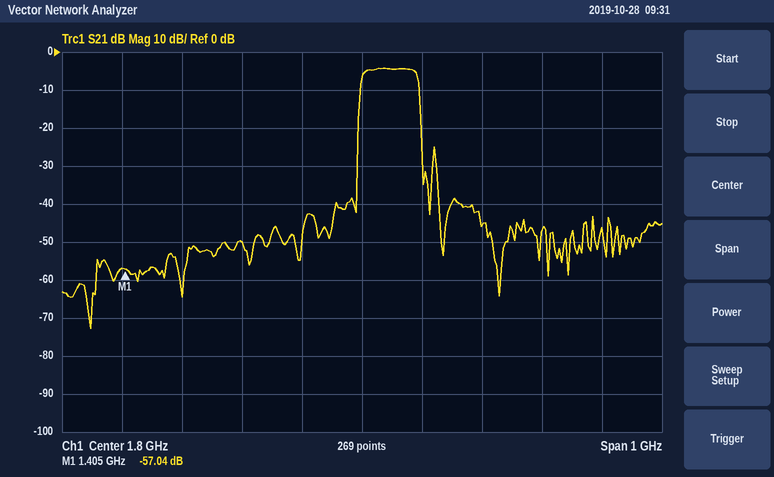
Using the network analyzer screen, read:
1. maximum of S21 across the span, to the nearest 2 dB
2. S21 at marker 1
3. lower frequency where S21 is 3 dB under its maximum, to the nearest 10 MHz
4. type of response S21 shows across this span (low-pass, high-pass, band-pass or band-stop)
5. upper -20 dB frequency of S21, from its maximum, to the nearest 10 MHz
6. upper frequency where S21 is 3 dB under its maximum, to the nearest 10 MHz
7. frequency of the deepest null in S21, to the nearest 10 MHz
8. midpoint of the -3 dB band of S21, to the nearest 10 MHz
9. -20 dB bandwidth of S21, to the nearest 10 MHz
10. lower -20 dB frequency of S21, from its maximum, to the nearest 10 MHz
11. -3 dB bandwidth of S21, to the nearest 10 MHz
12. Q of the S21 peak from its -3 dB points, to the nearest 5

-4 dB
-57.04 dB
1.80 GHz
band-pass
1.90 GHz
1.89 GHz
1.35 GHz
1.85 GHz
110 MHz
1.79 GHz
90 MHz
20
